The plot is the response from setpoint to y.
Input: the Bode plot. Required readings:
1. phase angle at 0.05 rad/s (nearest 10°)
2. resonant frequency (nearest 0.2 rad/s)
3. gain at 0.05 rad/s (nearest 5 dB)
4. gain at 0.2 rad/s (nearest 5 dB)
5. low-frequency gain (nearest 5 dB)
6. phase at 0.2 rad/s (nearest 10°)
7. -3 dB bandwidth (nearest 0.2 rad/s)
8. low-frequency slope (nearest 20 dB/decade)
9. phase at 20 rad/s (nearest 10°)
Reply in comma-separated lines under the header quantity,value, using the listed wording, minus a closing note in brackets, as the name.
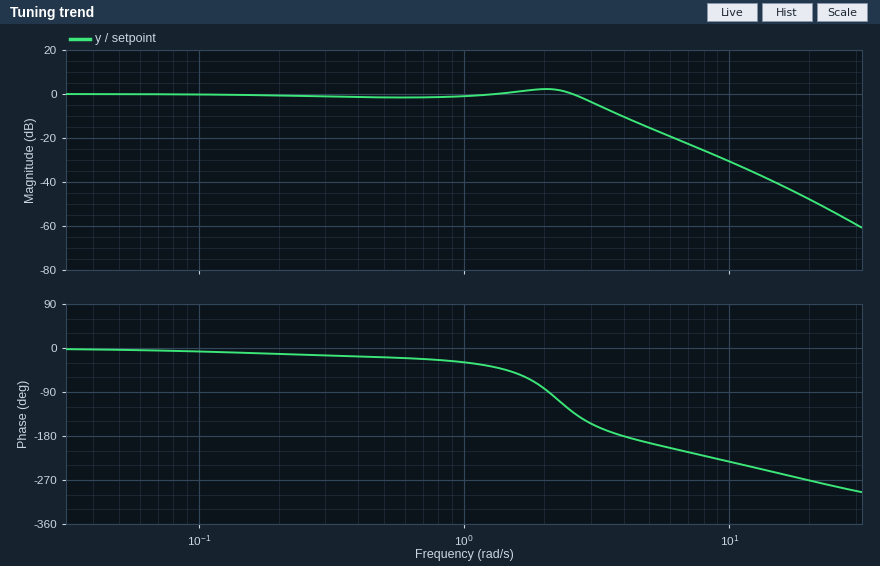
quantity,value
phase angle at 0.05 rad/s,0°
resonant frequency,2.0 rad/s
gain at 0.05 rad/s,0 dB
gain at 0.2 rad/s,0 dB
low-frequency gain,0 dB
phase at 0.2 rad/s,-10°
-3 dB bandwidth,3.0 rad/s
low-frequency slope,0 dB/decade
phase at 20 rad/s,-270°
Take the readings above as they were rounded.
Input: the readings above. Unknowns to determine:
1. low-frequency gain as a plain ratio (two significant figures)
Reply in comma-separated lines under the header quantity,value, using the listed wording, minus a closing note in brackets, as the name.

quantity,value
low-frequency gain as a plain ratio,1.0
